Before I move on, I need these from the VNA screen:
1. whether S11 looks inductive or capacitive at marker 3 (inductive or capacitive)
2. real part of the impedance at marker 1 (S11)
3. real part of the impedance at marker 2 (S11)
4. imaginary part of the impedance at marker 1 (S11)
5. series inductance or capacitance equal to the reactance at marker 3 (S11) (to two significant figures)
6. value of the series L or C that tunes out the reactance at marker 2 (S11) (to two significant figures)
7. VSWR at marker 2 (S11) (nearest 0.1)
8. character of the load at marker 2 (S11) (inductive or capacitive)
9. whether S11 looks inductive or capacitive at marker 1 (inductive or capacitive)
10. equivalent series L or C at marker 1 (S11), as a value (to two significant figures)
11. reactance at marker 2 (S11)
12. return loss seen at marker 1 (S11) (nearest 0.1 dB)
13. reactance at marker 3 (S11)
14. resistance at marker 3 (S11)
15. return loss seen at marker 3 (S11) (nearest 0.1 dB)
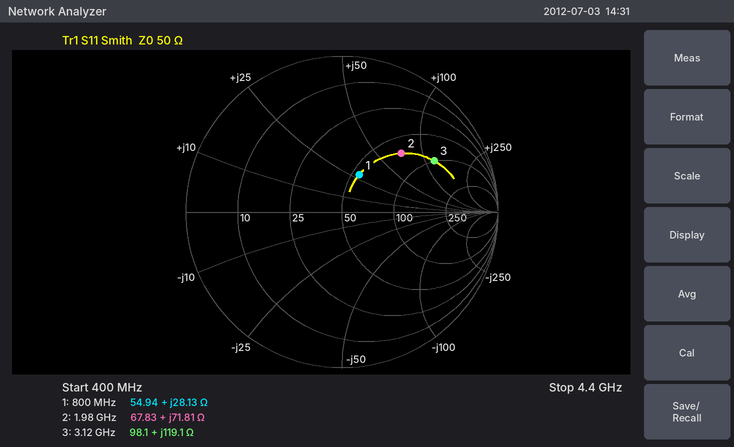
inductive
54.94 Ω
67.83 Ω
+28.13 Ω
6.1 nH
1.1 pF
3.3
inductive
inductive
5.6 nH
+71.81 Ω
11.6 dB
+119.1 Ω
98.1 Ω
3.4 dB
